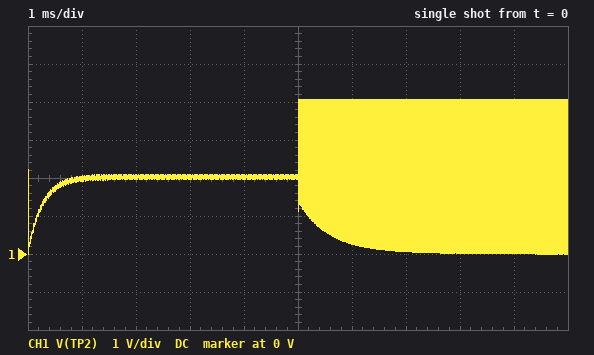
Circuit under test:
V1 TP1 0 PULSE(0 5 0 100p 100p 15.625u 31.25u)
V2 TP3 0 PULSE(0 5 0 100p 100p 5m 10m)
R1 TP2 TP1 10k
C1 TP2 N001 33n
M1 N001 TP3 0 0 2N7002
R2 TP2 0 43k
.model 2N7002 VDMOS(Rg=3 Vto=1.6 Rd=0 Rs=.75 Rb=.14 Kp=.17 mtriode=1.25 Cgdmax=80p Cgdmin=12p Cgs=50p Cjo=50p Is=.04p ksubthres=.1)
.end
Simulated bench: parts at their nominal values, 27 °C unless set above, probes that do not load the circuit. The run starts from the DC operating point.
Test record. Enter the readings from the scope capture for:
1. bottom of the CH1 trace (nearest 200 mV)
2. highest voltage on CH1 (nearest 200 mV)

0 V
4.0 V
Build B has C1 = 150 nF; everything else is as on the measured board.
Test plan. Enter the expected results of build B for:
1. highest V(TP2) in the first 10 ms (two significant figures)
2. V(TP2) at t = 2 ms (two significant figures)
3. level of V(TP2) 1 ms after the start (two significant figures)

4.1 V
1.6 V
1.1 V
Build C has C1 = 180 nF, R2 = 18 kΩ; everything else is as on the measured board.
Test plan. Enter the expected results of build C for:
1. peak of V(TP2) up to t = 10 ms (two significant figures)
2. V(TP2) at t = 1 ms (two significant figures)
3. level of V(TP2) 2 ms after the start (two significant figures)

3.2 V
920 mV
1.3 V
